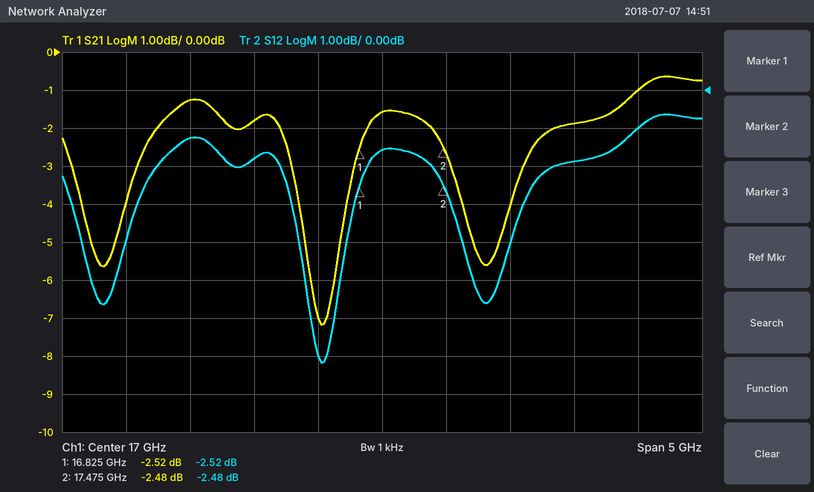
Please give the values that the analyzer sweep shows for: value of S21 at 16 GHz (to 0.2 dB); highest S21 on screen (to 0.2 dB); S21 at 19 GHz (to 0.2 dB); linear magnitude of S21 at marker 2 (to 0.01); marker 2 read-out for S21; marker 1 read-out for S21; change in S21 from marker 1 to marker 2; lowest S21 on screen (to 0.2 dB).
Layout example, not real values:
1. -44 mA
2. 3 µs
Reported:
1. -1.8 dB
2. -0.6 dB
3. -1.0 dB
4. 0.75
5. -2.48 dB
6. -2.52 dB
7. 0.04 dB
8. -7.2 dB
